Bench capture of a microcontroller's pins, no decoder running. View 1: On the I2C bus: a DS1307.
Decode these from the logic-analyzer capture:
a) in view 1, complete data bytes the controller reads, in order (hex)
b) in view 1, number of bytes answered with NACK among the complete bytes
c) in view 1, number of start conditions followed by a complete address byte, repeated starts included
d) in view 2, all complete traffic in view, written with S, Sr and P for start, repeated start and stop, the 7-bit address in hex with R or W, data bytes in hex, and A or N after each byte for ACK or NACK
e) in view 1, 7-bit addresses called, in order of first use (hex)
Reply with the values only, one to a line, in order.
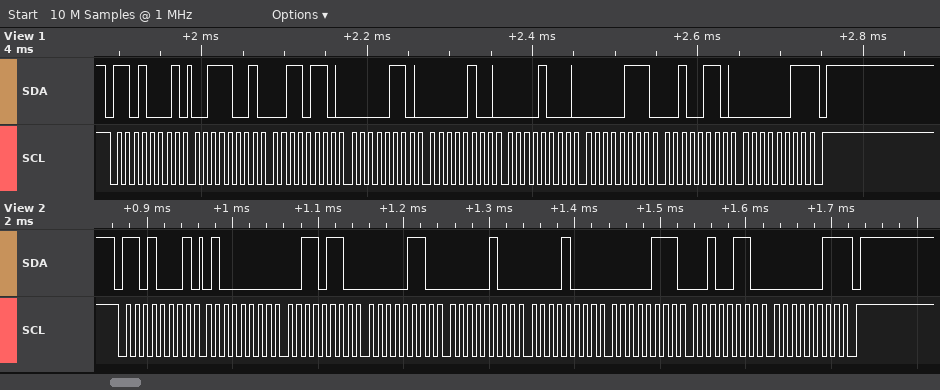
39 36 06 04 08 07 26 03
1
1
S 68R A 40 A 36 A 06 A 04 A 08 A 07 A 26 A 03 N P
0x68
